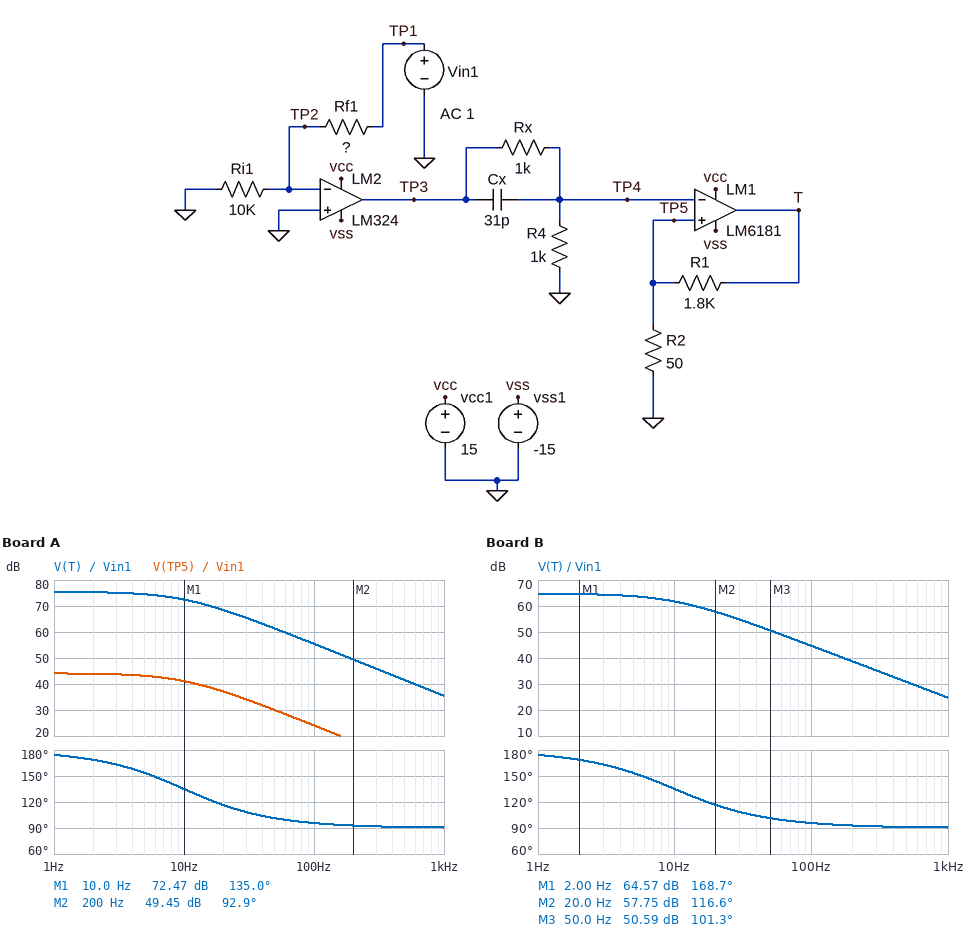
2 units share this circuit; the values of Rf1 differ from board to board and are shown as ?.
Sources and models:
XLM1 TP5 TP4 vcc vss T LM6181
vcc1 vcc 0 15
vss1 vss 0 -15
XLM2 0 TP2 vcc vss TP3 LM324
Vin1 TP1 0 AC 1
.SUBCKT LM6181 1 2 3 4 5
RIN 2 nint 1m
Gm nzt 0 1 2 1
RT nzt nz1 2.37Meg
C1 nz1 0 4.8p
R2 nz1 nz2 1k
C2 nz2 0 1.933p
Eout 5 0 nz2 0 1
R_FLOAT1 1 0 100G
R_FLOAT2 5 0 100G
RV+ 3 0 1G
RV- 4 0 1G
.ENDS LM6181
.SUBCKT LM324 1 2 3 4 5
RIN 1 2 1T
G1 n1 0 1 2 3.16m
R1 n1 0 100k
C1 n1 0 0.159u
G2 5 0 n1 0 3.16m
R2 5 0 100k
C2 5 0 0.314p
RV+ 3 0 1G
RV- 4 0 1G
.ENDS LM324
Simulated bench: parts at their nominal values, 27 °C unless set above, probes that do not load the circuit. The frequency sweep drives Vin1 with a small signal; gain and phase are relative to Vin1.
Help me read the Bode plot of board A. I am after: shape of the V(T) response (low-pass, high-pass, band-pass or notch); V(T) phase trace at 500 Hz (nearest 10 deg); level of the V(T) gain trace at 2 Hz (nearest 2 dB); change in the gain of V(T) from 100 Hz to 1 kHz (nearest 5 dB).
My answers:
low-pass
90 deg
76 dB
-20 dB
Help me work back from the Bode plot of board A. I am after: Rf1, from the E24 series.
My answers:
51 kΩ
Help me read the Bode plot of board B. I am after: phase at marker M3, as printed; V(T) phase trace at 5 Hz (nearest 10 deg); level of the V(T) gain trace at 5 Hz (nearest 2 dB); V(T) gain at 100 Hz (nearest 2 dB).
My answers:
101.3 deg
150 deg
64 dB
44 dB
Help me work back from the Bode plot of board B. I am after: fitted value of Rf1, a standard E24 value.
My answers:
200 kΩ
